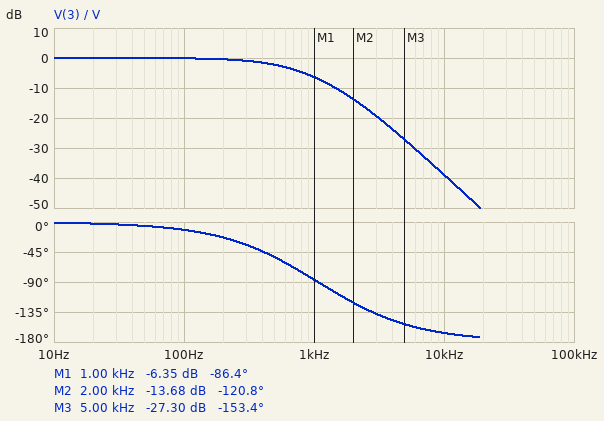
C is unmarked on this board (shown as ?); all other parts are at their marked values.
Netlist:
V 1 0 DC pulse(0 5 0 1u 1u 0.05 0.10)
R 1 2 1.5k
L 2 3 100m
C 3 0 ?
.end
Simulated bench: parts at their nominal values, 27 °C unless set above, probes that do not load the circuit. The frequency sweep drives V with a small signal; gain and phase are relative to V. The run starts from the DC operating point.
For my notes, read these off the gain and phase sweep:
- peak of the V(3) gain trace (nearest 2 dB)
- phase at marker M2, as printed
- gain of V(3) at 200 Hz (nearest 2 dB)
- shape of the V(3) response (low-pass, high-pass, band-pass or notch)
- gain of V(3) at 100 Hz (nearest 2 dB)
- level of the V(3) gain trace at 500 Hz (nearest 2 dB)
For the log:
0 dB
-120.8 deg
0 dB
low-pass
0 dB
-2 dB
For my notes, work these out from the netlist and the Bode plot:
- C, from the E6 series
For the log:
220 nF
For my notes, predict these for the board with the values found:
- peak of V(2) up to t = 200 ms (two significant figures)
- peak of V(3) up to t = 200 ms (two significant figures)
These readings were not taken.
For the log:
5.0 V
5.0 V
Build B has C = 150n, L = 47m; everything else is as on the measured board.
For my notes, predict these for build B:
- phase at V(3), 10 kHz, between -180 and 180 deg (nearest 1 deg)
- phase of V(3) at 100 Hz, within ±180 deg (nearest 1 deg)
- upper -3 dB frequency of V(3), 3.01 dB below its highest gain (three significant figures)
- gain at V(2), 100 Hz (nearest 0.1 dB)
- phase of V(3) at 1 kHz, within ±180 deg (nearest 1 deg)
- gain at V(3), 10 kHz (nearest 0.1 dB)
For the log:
-152 deg
-8 deg
818 Hz
-0.1 dB
-63 deg
-29.6 dB
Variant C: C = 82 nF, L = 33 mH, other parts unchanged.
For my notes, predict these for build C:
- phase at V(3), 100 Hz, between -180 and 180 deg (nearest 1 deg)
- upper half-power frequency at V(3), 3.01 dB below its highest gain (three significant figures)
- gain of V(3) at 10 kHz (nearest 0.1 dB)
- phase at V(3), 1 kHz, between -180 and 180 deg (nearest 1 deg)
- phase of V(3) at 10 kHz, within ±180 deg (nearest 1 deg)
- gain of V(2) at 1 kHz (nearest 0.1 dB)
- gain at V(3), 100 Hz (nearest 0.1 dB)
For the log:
-4 deg
1.56 kHz
-21.9 dB
-41 deg
-141 deg
-2.4 dB
0 dB
